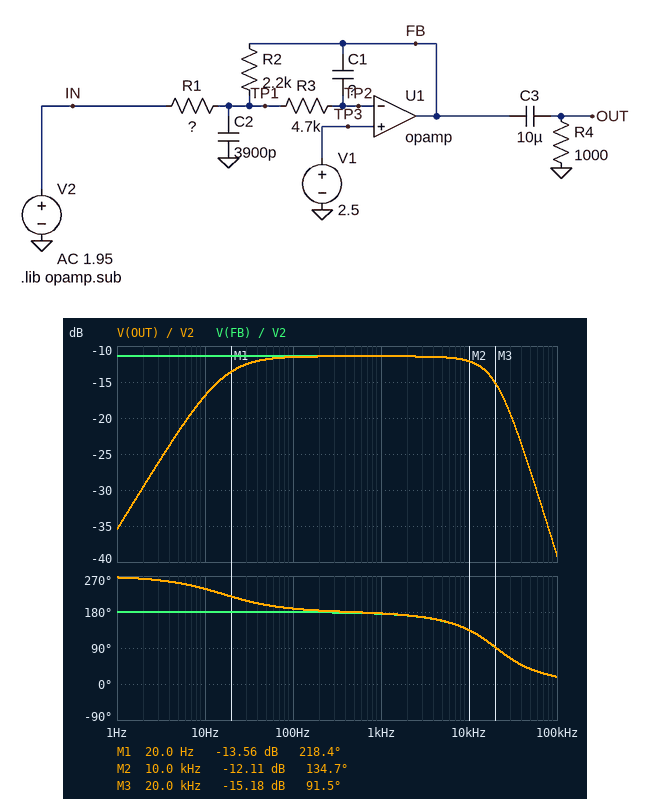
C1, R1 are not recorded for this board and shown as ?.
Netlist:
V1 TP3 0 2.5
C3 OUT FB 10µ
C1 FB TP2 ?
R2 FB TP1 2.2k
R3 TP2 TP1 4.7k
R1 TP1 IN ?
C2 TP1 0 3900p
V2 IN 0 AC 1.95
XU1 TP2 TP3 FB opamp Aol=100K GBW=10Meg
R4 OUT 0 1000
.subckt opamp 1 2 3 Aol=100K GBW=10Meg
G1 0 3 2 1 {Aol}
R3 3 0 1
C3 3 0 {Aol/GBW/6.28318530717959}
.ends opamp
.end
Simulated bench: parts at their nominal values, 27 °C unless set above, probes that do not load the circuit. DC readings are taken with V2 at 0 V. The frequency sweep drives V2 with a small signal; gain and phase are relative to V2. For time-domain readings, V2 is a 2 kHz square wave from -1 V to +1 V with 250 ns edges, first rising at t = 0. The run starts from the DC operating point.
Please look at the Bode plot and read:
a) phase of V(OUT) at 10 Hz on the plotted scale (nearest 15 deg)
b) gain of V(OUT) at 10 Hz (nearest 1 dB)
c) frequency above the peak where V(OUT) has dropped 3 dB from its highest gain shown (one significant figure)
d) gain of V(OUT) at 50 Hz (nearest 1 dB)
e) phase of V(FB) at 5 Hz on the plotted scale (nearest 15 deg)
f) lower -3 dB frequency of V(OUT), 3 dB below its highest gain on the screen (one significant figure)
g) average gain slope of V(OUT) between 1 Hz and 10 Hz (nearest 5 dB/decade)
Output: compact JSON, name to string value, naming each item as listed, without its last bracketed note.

{"phase of V(OUT) at 10 Hz on the plotted scale": "240 deg", "gain of V(OUT) at 10 Hz": "-17 dB", "frequency above the peak where V(OUT) has dropped 3 dB from its highest gain shown": "20 kHz", "gain of V(OUT) at 50 Hz": "-12 dB", "phase of V(FB) at 5 Hz on the plotted scale": "180 deg", "lower -3 dB frequency of V(OUT), 3 dB below its highest gain on the screen": "20 Hz", "average gain slope of V(OUT) between 1 Hz and 10 Hz": "20 dB/decade"}
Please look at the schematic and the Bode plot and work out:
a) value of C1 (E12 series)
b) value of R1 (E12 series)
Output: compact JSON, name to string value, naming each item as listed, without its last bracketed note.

{"value of C1": "1.5 nF", "value of R1": "8.2 kΩ"}
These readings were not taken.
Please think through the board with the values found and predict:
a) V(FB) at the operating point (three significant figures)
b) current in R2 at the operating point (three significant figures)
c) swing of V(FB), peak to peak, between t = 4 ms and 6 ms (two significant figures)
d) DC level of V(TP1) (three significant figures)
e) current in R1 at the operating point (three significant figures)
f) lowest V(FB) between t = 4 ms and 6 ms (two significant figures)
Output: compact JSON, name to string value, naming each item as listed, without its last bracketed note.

{"V(FB) at the operating point": "3.17 V", "current in R2 at the operating point": "305 µA", "swing of V(FB), peak to peak, between t = 4 ms and 6 ms": "560 mV", "DC level of V(TP1)": "2.50 V", "current in R1 at the operating point": "305 µA", "lowest V(FB) between t = 4 ms and 6 ms": "2.9 V"}
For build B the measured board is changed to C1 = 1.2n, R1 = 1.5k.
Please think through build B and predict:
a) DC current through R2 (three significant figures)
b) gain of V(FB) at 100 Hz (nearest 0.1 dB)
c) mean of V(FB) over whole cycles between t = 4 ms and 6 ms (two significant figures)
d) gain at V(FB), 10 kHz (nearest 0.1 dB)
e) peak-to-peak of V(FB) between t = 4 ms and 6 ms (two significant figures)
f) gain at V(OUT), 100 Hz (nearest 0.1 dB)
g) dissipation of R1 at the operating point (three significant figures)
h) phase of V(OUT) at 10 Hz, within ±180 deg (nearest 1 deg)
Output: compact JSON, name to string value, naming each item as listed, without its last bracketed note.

{"DC current through R2": "1.67 mA", "gain of V(FB) at 100 Hz": "3.3 dB", "mean of V(FB) over whole cycles between t = 4 ms and 6 ms": "6.2 V", "gain at V(FB), 10 kHz": "0.9 dB", "peak-to-peak of V(FB) between t = 4 ms and 6 ms": "2.9 V", "gain at V(OUT), 100 Hz": "3.2 dB", "dissipation of R1 at the operating point": "4.17 mW", "phase of V(OUT) at 10 Hz, within ±180 deg": "-122 deg"}
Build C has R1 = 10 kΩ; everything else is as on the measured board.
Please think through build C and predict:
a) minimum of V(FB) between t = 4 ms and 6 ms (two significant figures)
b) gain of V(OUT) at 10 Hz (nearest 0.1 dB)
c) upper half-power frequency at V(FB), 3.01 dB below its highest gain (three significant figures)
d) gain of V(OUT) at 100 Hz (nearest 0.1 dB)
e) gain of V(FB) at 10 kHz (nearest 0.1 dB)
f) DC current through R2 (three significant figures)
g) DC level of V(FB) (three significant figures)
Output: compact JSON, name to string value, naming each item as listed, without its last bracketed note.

{"minimum of V(FB) between t = 4 ms and 6 ms": "2.8 V", "gain of V(OUT) at 10 Hz": "-18.6 dB", "upper half-power frequency at V(FB), 3.01 dB below its highest gain": "18.8 kHz", "gain of V(OUT) at 100 Hz": "-13.3 dB", "gain of V(FB) at 10 kHz": "-13.7 dB", "DC current through R2": "250 µA", "DC level of V(FB)": "3.05 V"}
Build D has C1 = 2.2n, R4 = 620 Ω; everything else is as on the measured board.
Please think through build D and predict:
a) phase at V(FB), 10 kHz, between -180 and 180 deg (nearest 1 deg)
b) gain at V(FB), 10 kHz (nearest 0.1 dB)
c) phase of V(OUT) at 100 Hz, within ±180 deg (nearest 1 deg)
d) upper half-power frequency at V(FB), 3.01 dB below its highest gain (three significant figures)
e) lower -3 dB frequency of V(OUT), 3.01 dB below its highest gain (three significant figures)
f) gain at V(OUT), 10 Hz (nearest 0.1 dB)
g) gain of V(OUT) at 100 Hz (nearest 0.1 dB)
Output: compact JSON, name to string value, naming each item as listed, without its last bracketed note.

{"phase at V(FB), 10 kHz, between -180 and 180 deg": "120 deg", "gain at V(FB), 10 kHz": "-13.7 dB", "phase of V(OUT) at 100 Hz, within ±180 deg": "-166 deg", "upper half-power frequency at V(FB), 3.01 dB below its highest gain": "11.6 kHz", "lower -3 dB frequency of V(OUT), 3.01 dB below its highest gain": "25.6 Hz", "gain at V(OUT), 10 Hz": "-20.2 dB", "gain of V(OUT) at 100 Hz": "-11.7 dB"}
